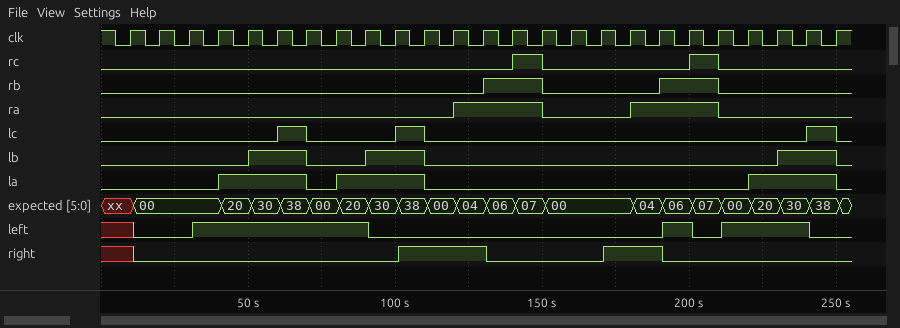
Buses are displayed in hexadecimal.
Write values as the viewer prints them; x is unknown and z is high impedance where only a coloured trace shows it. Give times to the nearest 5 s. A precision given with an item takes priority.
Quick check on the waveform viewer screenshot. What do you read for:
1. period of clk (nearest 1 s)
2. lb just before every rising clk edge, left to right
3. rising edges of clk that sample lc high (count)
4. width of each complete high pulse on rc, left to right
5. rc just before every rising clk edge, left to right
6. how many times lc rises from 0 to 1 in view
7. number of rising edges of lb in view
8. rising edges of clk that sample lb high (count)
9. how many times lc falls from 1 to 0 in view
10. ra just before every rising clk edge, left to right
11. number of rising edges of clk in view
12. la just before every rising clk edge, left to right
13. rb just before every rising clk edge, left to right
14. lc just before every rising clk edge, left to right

10 s
0 0 0 0 0 1 1 0 0 1 1 0 0 0 0 0 0 0 0 0 0 0 0 1 1
3
10 s, 10 s
0 0 0 0 0 0 0 0 0 0 0 0 0 0 1 0 0 0 0 0 1 0 0 0 0
3
3
6
3
0 0 0 0 0 0 0 0 0 0 0 0 1 1 1 0 0 0 1 1 1 0 0 0 0
25
0 0 0 0 1 1 1 0 1 1 1 0 0 0 0 0 0 0 0 0 0 0 1 1 1
0 0 0 0 0 0 0 0 0 0 0 0 0 1 1 0 0 0 0 1 1 0 0 0 0
0 0 0 0 0 0 1 0 0 0 1 0 0 0 0 0 0 0 0 0 0 0 0 0 1
